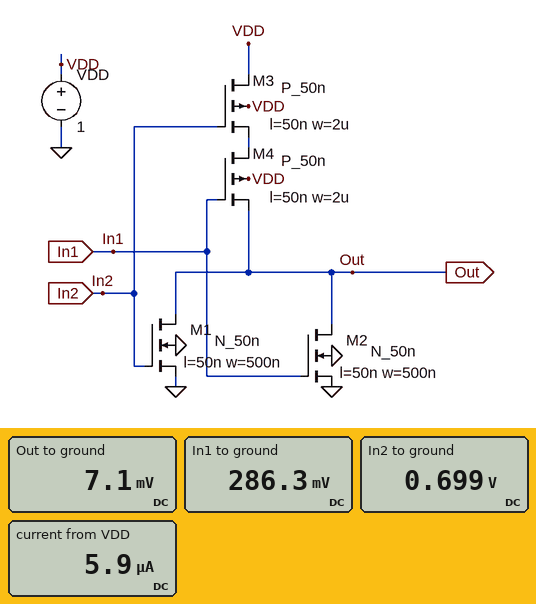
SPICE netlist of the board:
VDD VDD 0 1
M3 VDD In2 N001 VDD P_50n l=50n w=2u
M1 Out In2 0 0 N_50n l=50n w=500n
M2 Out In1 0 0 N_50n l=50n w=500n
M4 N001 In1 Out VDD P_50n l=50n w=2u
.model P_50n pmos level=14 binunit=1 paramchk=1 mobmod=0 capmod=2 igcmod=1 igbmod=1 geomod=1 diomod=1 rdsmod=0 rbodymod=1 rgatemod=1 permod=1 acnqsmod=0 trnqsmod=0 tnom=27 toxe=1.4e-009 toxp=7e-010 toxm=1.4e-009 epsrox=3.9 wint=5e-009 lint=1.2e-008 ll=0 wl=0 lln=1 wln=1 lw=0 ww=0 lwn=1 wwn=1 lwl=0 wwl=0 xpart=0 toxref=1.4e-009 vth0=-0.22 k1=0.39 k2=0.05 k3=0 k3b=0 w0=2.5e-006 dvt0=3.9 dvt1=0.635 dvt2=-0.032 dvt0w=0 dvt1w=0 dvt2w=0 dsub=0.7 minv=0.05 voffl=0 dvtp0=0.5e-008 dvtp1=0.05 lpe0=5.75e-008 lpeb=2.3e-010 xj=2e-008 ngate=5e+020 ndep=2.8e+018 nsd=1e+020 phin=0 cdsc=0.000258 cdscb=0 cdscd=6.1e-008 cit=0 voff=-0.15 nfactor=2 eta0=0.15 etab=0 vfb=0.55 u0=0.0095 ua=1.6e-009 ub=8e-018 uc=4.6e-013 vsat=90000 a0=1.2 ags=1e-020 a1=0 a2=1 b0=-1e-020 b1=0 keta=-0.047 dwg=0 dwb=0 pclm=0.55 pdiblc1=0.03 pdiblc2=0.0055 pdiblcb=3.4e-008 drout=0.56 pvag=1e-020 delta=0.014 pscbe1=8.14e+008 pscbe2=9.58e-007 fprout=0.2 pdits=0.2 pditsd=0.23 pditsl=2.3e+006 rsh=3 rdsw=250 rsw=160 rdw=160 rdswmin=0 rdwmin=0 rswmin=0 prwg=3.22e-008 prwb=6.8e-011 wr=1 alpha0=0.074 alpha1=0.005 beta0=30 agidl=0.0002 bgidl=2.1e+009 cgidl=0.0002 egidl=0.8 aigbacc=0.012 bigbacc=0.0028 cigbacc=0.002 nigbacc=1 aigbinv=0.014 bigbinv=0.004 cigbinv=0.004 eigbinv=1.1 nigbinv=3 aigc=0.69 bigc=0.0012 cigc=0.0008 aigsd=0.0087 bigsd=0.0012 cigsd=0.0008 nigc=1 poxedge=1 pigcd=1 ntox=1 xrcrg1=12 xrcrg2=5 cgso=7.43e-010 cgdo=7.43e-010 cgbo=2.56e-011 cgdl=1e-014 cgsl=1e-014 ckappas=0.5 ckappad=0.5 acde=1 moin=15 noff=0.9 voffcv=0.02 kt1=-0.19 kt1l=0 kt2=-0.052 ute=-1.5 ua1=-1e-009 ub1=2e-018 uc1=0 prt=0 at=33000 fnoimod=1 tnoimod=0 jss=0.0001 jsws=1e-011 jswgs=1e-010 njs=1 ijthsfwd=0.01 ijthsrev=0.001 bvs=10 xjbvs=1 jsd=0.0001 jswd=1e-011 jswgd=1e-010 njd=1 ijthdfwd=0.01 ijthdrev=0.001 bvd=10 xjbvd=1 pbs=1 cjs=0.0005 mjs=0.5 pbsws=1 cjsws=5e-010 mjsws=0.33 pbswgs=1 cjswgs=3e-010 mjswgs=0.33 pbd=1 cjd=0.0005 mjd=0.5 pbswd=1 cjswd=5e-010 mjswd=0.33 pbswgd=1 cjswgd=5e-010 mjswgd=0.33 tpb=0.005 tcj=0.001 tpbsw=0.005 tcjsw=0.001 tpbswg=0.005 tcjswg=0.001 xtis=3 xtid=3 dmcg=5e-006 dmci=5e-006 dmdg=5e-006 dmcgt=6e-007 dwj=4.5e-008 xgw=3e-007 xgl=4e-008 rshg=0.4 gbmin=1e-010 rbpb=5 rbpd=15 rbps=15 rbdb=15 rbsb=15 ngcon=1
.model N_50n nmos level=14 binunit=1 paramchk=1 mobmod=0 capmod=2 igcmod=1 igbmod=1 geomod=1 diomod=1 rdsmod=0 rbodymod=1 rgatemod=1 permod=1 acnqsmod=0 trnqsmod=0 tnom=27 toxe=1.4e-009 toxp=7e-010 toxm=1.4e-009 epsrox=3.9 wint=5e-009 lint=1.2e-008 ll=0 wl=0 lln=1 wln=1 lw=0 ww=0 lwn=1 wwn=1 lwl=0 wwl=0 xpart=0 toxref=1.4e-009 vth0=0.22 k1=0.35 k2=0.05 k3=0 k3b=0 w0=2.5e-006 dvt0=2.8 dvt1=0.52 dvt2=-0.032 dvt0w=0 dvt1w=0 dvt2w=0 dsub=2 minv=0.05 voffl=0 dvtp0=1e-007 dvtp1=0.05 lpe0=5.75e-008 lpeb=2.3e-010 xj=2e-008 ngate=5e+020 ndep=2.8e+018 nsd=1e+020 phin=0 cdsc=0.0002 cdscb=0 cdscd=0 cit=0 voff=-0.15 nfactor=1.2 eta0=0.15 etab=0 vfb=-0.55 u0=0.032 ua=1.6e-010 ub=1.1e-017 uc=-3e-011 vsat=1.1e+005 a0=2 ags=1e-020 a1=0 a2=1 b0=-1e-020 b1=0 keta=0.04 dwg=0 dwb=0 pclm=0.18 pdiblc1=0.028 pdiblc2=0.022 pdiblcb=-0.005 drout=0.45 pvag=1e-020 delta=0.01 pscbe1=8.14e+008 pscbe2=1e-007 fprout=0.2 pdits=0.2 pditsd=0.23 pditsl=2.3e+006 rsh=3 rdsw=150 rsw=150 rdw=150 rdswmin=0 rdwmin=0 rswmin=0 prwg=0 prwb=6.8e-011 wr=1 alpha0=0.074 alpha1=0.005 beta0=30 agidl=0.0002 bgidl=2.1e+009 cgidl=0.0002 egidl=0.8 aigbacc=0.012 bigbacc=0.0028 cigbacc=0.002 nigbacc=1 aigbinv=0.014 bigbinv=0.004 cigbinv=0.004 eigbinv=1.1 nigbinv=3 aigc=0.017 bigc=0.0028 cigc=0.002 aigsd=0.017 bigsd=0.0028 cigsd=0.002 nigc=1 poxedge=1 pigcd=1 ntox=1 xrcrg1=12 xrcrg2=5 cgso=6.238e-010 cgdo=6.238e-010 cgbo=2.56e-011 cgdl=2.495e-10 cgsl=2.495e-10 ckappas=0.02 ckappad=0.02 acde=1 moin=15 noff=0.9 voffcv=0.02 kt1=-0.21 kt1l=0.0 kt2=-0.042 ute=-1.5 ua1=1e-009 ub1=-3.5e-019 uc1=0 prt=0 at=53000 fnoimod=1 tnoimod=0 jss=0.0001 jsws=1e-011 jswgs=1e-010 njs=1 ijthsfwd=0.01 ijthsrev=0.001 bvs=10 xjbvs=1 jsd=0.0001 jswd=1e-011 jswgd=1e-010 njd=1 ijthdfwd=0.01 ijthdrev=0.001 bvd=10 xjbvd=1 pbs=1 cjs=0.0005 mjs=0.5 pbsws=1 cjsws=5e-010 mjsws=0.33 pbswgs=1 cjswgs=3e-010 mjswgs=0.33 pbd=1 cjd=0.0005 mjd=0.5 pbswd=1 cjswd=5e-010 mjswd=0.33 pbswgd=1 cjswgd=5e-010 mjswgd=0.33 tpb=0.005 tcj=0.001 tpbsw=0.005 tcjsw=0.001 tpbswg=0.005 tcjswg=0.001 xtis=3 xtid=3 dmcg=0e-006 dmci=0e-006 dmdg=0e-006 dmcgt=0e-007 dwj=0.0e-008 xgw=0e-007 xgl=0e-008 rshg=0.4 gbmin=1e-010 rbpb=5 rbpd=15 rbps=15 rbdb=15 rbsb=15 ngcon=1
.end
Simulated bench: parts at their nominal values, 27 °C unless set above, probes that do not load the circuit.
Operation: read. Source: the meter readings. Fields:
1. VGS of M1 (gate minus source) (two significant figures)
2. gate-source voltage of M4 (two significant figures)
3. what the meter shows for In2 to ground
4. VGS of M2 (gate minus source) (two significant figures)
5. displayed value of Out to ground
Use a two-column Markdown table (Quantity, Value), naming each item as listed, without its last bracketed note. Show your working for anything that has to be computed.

| Quantity | Value |
|---|---|
| VGS of M1 (gate minus source) | 699 mV = 700 mV |
| gate-source voltage of M4 | 286.3 mV - 7.1 mV = 280 mV |
| what the meter shows for In2 to ground | 0.699 V |
| VGS of M2 (gate minus source) | 286.3 mV = 290 mV |
| displayed value of Out to ground | 7.1 mV |
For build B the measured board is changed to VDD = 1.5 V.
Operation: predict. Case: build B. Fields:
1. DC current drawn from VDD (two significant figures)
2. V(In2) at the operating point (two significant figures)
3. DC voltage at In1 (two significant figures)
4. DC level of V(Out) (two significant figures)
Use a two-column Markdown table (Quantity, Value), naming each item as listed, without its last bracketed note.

| Quantity | Value |
|---|---|
| DC current drawn from VDD | 89 µA |
| V(In2) at the operating point | 1.0 V |
| DC voltage at In1 | 520 mV |
| DC level of V(Out) | 67 mV |
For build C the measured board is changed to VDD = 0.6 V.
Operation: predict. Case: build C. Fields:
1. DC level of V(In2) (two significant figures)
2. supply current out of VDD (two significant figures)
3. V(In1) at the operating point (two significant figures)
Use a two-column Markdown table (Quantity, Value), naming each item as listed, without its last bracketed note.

| Quantity | Value |
|---|---|
| DC level of V(In2) | 430 mV |
| supply current out of VDD | 320 nA |
| V(In1) at the operating point | 150 mV |
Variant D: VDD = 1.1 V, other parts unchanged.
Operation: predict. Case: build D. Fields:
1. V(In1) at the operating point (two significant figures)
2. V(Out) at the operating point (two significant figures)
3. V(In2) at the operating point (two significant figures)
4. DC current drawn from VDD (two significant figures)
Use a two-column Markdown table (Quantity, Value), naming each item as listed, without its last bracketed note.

| Quantity | Value |
|---|---|
| V(In1) at the operating point | 330 mV |
| V(Out) at the operating point | 13 mV |
| V(In2) at the operating point | 760 mV |
| DC current drawn from VDD | 12 µA |
